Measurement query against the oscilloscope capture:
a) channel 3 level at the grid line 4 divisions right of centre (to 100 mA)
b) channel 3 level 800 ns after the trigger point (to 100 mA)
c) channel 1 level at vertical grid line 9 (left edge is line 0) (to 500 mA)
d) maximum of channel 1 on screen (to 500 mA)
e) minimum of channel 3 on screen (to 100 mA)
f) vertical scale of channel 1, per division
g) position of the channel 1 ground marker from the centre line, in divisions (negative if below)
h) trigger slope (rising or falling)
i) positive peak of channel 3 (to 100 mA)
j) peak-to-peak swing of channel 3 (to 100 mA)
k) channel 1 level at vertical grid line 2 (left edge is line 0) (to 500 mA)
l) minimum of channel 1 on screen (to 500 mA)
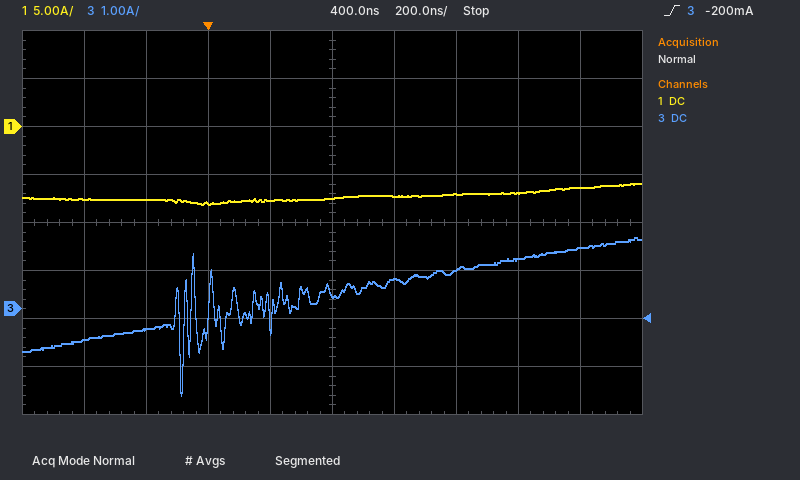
1.3 A
800 mA
-6.5 A
-6.0 A
-1.8 A
5 A
+2.0 div
rising
1.5 A
3.3 A
-7.5 A
-8.0 A
